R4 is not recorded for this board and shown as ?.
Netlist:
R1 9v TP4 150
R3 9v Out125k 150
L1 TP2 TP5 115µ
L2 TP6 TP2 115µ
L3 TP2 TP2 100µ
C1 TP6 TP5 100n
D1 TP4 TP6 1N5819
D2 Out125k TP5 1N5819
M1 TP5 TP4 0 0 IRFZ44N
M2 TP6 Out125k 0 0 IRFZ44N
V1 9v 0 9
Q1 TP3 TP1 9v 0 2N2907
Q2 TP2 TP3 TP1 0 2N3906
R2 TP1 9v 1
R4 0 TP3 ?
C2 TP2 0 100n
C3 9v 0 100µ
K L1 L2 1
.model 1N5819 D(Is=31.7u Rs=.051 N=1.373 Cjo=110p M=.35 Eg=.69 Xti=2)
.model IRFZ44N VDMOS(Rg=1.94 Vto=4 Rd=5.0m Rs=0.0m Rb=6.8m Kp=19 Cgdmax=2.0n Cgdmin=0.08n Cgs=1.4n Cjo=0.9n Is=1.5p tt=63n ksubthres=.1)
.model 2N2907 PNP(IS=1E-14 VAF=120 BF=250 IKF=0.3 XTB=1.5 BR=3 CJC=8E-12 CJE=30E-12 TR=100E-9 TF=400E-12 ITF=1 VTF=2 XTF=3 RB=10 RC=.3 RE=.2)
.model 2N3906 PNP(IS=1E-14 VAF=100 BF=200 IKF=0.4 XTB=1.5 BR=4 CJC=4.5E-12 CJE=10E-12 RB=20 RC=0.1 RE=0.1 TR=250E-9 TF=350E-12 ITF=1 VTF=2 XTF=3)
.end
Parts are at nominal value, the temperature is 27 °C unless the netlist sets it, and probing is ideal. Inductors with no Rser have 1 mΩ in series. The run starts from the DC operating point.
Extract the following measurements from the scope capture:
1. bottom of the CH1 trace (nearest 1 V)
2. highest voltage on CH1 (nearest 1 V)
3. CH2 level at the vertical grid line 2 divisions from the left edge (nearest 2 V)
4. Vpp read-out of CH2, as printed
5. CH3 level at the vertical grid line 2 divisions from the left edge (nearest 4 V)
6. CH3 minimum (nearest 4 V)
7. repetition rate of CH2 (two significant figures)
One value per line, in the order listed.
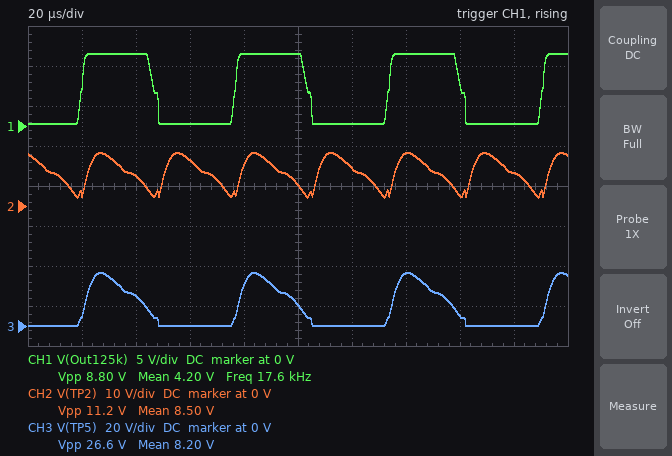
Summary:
0 V
9 V
8 V
11.2 V
16 V
0 V
35 kHz
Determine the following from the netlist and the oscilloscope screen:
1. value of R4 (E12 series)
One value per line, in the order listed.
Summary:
1.5 kΩ
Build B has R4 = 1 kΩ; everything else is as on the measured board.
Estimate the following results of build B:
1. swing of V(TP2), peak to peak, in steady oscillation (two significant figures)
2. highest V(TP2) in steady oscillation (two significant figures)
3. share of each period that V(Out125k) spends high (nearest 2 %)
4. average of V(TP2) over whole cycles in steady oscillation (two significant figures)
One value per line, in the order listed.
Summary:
12 V
14 V
46 %
8.7 V
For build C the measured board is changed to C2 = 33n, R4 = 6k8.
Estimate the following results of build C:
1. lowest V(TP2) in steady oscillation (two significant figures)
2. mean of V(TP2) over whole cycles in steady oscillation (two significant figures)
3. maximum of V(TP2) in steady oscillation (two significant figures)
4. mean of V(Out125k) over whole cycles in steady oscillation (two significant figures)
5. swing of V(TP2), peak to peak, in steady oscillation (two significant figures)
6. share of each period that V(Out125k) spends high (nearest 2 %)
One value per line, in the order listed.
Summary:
2.0 V
7.7 V
12 V
4.3 V
9.9 V
44 %
